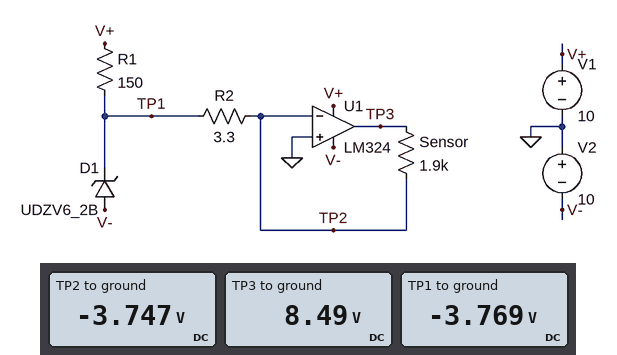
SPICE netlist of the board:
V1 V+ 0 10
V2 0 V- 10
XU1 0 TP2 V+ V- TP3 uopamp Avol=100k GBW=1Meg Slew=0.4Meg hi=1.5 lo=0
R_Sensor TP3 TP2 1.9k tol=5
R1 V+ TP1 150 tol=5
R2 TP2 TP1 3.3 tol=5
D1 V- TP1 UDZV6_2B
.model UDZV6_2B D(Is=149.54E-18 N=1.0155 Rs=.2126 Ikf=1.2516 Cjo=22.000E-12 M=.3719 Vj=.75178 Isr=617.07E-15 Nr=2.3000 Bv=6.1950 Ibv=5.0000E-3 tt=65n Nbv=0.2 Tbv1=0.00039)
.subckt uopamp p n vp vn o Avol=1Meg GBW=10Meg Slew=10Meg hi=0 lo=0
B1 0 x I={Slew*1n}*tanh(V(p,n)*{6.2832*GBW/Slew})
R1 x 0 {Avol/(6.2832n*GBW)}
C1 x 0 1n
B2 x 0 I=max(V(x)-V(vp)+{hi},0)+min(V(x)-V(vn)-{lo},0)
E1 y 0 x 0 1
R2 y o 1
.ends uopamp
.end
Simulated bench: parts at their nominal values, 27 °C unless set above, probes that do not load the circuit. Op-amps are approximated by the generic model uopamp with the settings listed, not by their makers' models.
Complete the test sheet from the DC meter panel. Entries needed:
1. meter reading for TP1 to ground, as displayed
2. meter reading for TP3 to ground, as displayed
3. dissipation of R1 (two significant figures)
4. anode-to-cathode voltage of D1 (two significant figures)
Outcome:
-3.769 V
8.49 V
1.3 W
-6.2 V
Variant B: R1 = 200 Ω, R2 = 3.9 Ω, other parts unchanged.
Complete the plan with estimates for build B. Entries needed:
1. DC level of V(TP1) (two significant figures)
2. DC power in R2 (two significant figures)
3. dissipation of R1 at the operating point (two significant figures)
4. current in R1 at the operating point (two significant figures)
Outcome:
-3.8 V
160 µW
950 mW
69 mA
